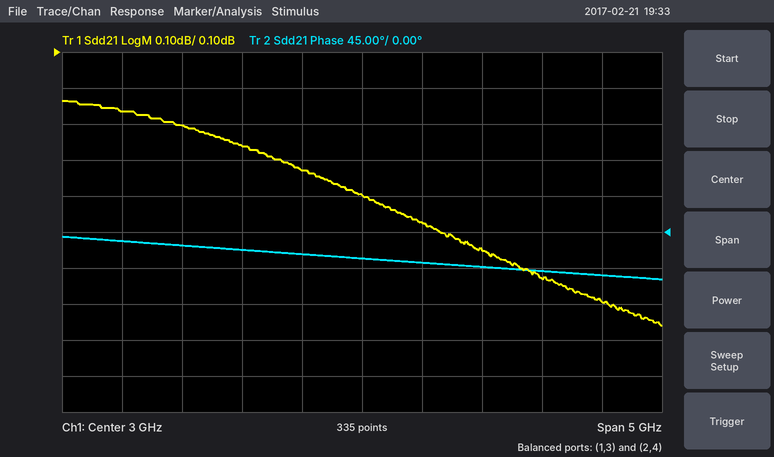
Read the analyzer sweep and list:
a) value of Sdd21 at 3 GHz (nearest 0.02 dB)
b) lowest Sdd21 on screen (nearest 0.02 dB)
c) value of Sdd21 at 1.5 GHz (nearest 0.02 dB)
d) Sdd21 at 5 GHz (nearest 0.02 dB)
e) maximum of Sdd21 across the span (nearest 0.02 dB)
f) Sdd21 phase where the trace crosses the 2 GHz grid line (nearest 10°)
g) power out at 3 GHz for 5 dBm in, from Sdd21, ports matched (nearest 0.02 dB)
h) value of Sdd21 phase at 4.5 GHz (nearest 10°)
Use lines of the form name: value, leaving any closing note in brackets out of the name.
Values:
value of Sdd21 at 3 GHz: -0.30 dB
lowest Sdd21 on screen: -0.66 dB
value of Sdd21 at 1.5 GHz: -0.10 dB
Sdd21 at 5 GHz: -0.60 dB
maximum of Sdd21 across the span: -0.04 dB
Sdd21 phase where the trace crosses the 2 GHz grid line: -20°
power out at 3 GHz for 5 dBm in, from Sdd21, ports matched: 4.70 dBm
value of Sdd21 phase at 4.5 GHz: -50°
